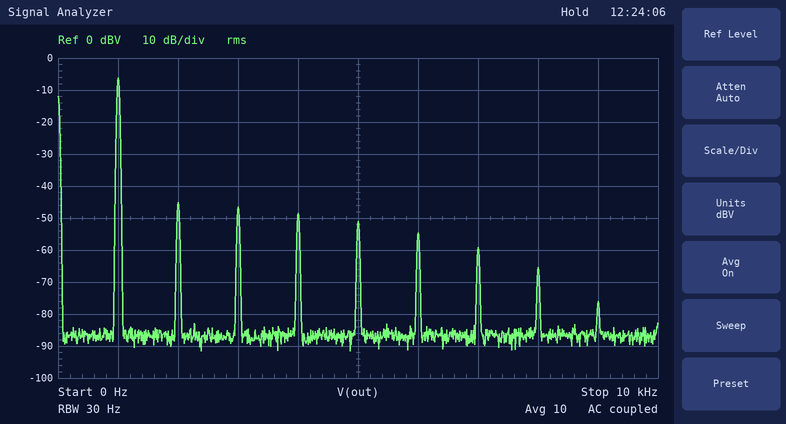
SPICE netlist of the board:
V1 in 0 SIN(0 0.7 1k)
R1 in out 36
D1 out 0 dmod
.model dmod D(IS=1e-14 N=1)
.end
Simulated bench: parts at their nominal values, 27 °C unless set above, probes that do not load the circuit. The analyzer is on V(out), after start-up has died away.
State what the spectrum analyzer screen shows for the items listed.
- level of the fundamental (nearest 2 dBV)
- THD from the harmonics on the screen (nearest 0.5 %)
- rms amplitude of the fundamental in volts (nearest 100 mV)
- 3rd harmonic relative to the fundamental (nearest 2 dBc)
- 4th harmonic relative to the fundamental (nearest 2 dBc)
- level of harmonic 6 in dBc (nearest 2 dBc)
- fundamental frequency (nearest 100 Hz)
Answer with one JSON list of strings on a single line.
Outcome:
["-6 dBV", "2.0 %", "500 mV", "-40 dBc", "-42 dBc", "-48 dBc", "1.0 kHz"]
